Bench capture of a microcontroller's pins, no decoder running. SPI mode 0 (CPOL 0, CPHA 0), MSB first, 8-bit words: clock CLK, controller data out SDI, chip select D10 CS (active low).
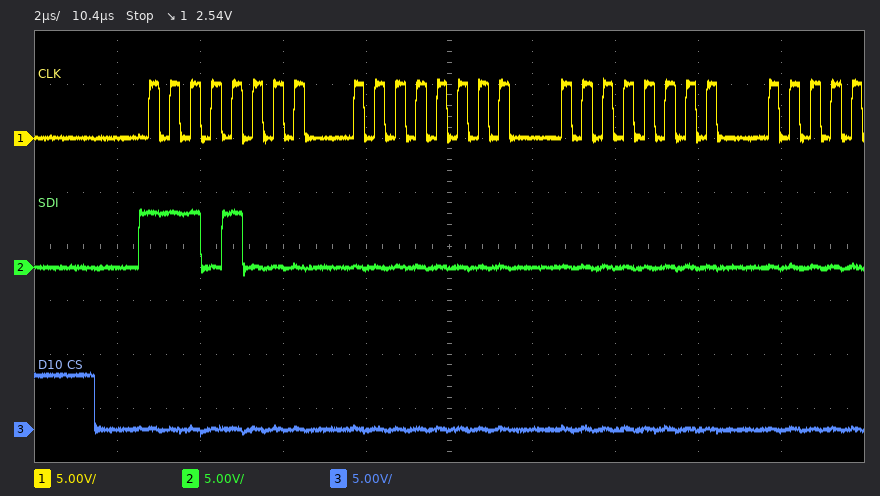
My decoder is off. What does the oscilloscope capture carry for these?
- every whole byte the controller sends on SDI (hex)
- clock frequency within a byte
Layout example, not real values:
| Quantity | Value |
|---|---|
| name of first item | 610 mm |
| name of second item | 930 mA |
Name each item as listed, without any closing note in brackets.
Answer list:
| Quantity | Value |
|---|---|
| every whole byte the controller sends on SDI | E8 00 00 |
| clock frequency within a byte | 2 MHz |
